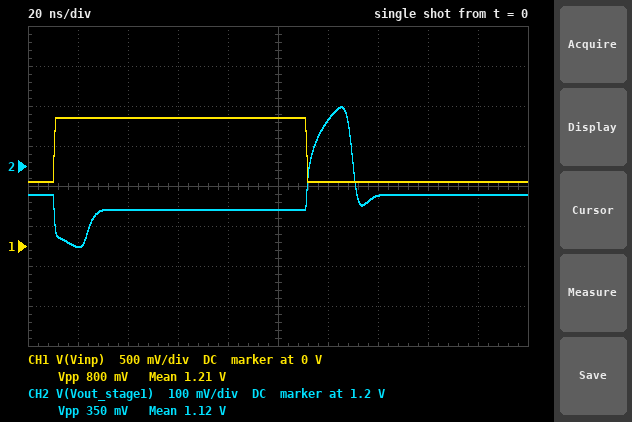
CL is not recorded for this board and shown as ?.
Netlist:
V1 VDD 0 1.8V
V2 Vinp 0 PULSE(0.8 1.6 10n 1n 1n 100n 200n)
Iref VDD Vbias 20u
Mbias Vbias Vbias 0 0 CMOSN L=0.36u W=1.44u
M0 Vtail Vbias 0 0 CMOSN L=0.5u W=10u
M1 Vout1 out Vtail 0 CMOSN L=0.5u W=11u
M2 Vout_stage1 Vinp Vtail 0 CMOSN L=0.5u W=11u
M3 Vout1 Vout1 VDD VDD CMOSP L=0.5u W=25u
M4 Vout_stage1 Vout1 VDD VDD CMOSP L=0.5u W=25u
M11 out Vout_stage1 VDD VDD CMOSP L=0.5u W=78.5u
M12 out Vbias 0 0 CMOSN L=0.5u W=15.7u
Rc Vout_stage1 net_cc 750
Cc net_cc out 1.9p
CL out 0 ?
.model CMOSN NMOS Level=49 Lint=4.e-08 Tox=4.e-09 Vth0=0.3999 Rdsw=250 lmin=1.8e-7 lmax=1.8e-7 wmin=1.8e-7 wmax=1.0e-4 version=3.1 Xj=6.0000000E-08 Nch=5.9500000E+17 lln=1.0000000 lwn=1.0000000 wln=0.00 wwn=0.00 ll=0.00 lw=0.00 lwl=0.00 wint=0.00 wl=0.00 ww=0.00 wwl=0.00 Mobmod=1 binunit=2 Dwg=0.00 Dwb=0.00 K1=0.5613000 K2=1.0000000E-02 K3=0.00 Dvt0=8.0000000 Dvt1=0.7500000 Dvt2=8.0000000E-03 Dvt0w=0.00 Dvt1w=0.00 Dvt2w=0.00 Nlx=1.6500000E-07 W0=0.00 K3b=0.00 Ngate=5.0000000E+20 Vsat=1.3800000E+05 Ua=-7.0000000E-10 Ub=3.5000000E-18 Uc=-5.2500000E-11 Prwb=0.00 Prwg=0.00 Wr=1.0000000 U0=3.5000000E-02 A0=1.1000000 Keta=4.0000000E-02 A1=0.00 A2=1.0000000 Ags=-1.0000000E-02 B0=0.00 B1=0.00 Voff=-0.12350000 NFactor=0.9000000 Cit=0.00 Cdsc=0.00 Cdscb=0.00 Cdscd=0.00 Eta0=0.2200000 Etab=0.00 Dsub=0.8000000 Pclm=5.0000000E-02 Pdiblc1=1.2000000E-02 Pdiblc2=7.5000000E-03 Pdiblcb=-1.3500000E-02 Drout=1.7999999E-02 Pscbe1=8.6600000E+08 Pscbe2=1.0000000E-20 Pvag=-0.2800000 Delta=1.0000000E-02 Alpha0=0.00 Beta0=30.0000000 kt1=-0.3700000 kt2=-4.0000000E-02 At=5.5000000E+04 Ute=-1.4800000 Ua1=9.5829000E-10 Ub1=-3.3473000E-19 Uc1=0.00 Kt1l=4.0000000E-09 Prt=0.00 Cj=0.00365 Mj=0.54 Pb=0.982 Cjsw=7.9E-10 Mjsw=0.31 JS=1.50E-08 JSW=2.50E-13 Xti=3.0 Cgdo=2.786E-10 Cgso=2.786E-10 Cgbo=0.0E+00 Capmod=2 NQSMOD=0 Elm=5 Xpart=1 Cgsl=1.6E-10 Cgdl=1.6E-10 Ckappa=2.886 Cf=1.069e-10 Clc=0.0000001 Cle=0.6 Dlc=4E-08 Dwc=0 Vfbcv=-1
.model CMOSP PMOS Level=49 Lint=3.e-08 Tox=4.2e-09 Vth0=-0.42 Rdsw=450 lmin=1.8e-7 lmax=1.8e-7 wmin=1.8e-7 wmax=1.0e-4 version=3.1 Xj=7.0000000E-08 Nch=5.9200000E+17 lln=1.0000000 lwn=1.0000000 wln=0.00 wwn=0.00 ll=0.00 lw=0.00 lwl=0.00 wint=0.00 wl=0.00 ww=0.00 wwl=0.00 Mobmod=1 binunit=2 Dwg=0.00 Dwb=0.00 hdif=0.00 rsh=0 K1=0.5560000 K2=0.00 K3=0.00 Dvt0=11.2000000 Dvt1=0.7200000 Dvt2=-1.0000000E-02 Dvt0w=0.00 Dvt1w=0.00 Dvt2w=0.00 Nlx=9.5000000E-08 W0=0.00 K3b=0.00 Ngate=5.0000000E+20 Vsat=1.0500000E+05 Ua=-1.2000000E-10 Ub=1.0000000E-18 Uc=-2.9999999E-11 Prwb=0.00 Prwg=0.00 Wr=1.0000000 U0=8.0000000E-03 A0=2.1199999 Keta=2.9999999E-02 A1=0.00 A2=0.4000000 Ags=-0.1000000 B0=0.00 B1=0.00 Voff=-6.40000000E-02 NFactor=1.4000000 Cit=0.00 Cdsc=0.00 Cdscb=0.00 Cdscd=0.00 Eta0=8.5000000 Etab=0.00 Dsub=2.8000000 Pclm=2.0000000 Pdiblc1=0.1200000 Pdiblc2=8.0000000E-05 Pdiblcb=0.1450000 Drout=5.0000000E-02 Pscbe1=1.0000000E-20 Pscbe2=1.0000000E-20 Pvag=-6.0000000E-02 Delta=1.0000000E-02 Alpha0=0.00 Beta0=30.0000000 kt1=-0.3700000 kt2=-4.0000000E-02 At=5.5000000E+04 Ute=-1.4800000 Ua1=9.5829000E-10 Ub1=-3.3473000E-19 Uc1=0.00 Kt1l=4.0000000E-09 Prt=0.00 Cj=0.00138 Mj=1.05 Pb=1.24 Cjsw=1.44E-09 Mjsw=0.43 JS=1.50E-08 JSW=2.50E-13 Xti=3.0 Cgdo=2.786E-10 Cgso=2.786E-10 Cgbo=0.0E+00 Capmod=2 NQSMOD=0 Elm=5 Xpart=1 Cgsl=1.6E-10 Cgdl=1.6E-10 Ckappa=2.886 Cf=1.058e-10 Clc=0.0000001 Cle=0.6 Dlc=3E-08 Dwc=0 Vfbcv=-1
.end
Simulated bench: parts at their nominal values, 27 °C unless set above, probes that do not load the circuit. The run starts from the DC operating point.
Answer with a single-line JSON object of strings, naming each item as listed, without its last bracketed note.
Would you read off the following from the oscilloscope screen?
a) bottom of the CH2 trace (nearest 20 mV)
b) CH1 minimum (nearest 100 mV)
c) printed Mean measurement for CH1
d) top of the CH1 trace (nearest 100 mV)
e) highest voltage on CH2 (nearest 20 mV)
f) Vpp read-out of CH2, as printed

{"bottom of the CH2 trace": "1.00 V", "CH1 minimum": "800 mV", "printed Mean measurement for CH1": "1.21 V", "top of the CH1 trace": "1.6 V", "highest voltage on CH2": "1.34 V", "Vpp read-out of CH2, as printed": "350 mV"}
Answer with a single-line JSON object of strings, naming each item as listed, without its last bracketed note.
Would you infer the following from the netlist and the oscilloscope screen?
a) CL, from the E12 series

{"CL, from the E12 series": "1.8 pF"}
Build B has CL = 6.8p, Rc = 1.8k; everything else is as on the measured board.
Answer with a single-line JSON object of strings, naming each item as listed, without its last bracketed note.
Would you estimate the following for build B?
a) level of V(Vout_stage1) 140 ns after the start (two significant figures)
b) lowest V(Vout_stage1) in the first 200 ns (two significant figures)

{"level of V(Vout_stage1) 140 ns after the start": "1.7 V", "lowest V(Vout_stage1) in the first 200 ns": "890 mV"}
